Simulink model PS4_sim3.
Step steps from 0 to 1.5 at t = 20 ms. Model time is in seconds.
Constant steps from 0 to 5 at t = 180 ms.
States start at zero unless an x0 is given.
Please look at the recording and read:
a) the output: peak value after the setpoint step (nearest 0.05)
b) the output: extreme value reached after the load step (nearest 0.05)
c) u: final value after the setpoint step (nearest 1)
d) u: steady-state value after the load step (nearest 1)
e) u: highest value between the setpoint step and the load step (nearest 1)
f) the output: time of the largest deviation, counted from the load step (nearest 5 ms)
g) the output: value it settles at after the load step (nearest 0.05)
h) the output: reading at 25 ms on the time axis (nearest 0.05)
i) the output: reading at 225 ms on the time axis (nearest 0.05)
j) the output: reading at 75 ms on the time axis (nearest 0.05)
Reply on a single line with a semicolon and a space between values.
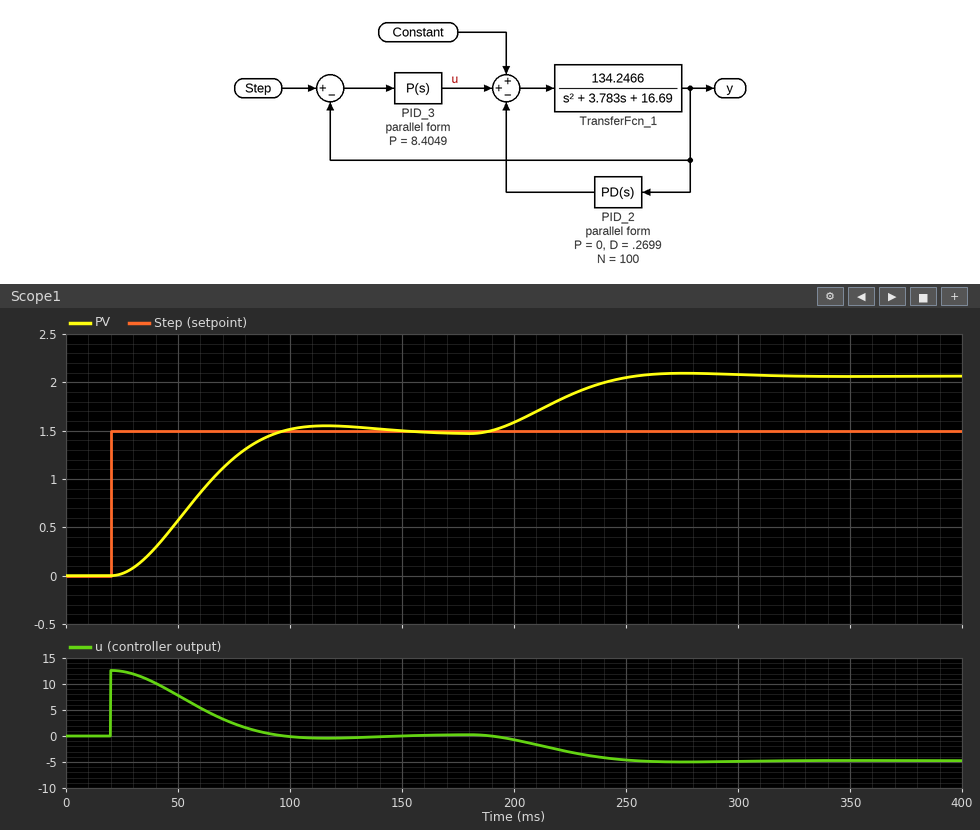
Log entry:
1.55; 2.10; 0; -5; 13; 95 ms; 2.05; 0.00; 1.85; 1.20
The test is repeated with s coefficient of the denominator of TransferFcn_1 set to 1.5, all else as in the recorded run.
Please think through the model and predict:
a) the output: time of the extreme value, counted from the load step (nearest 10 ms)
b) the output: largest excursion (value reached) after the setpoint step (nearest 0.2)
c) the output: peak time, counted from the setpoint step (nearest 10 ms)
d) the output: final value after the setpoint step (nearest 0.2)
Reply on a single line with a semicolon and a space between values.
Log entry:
90 ms; 1.6; 90 ms; 1.4
